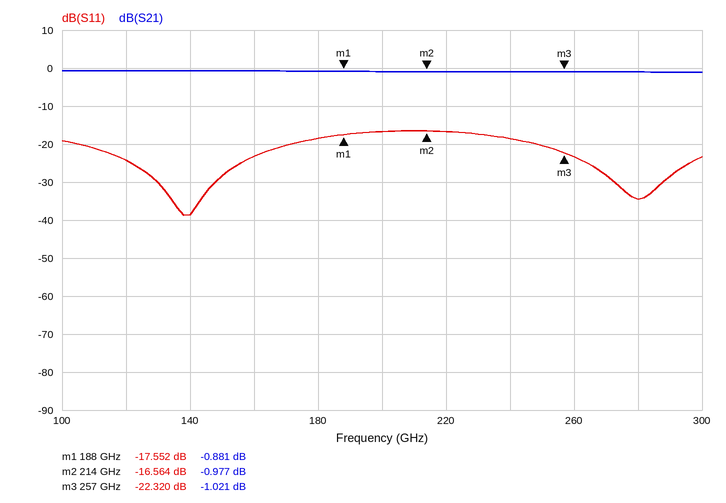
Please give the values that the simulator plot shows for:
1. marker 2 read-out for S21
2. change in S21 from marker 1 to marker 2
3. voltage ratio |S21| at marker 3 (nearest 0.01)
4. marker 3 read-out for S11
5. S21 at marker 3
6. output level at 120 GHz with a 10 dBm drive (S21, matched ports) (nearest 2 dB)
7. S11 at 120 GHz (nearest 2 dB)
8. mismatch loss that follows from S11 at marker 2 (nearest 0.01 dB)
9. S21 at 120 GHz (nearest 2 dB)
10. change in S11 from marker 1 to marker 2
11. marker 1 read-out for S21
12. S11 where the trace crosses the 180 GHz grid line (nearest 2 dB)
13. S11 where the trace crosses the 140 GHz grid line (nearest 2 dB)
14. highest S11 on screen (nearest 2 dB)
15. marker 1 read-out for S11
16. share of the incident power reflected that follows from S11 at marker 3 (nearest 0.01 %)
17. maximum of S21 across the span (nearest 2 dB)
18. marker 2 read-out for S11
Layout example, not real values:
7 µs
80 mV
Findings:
-0.977 dB
-0.096 dB
0.89
-22.320 dB
-1.021 dB
10 dBm
-24 dB
0.10 dB
0 dB
0.988 dB
-0.881 dB
-18 dB
-38 dB
-16 dB
-17.552 dB
0.59 %
0 dB
-16.564 dB
